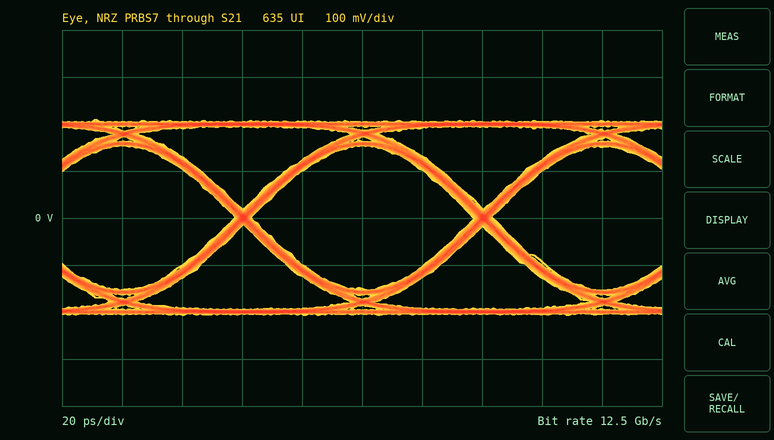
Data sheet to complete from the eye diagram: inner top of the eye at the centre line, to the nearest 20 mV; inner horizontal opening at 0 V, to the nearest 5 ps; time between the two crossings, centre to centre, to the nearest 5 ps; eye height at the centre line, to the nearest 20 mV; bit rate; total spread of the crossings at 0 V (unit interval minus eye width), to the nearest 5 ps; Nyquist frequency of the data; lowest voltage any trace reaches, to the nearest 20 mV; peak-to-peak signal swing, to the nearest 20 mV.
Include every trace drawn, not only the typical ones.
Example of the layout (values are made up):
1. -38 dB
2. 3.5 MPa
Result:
1. 160 mV
2. 75 ps
3. 80 ps
4. 300 mV
5. 12.5 Gb/s
6. 5 ps
7. 6.25 GHz
8. -200 mV
9. 420 mV
